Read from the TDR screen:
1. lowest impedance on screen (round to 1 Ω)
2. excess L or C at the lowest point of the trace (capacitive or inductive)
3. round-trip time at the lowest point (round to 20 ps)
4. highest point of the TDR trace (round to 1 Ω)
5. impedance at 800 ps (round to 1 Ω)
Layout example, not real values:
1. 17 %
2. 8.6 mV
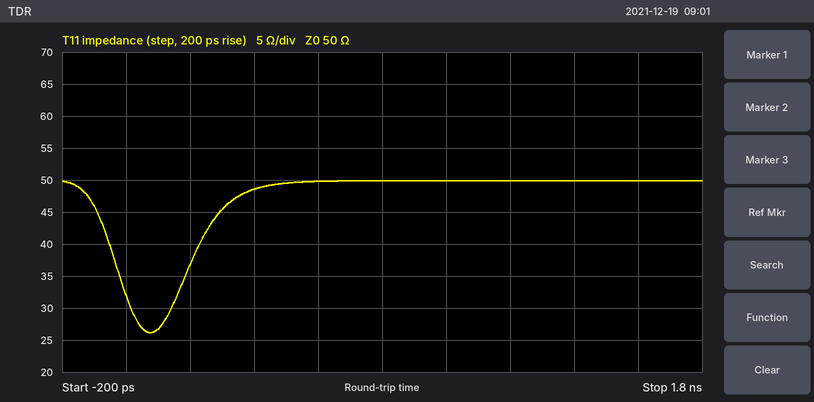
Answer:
1. 26 Ω
2. capacitive
3. 80 ps
4. 50 Ω
5. 50 Ω
